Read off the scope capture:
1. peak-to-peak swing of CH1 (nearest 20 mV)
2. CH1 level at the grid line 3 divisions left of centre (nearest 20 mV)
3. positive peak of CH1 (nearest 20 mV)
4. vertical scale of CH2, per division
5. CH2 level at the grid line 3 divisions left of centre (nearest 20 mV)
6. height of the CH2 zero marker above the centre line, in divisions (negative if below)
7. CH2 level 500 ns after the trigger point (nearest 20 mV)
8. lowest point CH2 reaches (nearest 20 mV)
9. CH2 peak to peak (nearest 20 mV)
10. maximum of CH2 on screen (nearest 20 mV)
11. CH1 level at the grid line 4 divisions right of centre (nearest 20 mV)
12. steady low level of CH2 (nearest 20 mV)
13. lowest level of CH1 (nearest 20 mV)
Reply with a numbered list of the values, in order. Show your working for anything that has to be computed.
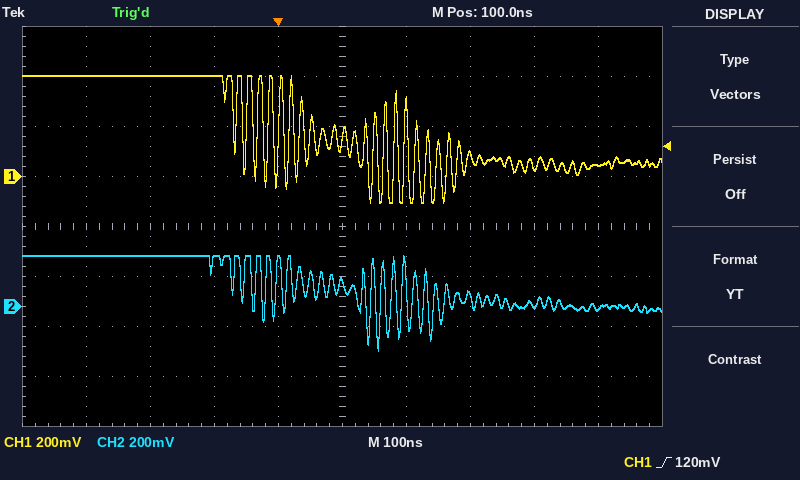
1. 400 mV − (-100 mV) = 500 mV
2. 400 mV
3. 400 mV
4. 200 mV
5. 200 mV
6. -1.6 div
7. 0 mV
8. -180 mV
9. 200 mV − (-180 mV) = 380 mV
10. 200 mV
11. 40 mV
12. 0 mV
13. -100 mV
